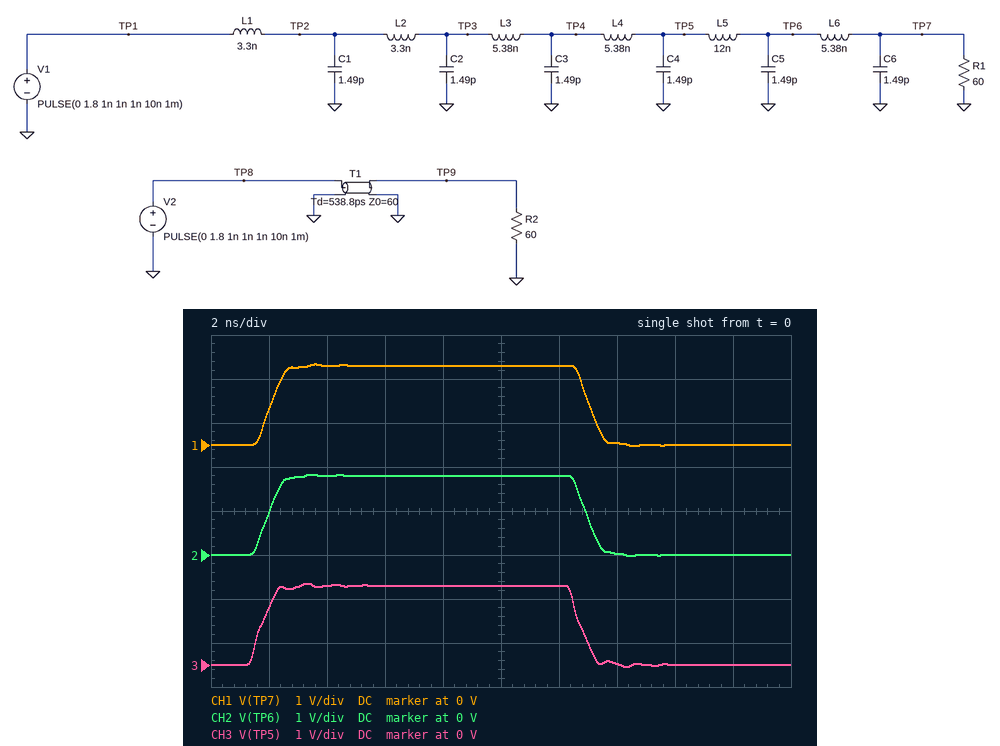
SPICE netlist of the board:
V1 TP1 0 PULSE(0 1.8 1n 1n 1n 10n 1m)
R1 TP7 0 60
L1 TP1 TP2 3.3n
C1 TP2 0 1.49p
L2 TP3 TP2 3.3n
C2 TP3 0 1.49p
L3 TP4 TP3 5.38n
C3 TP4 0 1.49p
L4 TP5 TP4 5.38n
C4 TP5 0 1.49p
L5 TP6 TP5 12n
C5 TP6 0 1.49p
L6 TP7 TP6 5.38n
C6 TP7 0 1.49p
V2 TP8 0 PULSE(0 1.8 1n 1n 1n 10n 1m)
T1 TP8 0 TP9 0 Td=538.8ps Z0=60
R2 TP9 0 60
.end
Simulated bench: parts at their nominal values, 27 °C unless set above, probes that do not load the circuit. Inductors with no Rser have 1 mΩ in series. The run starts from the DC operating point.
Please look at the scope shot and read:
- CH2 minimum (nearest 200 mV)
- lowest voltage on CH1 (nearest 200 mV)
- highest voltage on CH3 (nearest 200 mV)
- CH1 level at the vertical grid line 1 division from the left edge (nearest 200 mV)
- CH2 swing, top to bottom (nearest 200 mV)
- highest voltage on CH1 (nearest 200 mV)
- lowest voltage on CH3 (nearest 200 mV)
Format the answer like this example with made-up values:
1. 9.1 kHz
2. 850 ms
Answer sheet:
1. 0 V
2. 0 V
3. 1.8 V
4. 800 mV
5. 1.8 V
6. 1.8 V
7. 0 V
